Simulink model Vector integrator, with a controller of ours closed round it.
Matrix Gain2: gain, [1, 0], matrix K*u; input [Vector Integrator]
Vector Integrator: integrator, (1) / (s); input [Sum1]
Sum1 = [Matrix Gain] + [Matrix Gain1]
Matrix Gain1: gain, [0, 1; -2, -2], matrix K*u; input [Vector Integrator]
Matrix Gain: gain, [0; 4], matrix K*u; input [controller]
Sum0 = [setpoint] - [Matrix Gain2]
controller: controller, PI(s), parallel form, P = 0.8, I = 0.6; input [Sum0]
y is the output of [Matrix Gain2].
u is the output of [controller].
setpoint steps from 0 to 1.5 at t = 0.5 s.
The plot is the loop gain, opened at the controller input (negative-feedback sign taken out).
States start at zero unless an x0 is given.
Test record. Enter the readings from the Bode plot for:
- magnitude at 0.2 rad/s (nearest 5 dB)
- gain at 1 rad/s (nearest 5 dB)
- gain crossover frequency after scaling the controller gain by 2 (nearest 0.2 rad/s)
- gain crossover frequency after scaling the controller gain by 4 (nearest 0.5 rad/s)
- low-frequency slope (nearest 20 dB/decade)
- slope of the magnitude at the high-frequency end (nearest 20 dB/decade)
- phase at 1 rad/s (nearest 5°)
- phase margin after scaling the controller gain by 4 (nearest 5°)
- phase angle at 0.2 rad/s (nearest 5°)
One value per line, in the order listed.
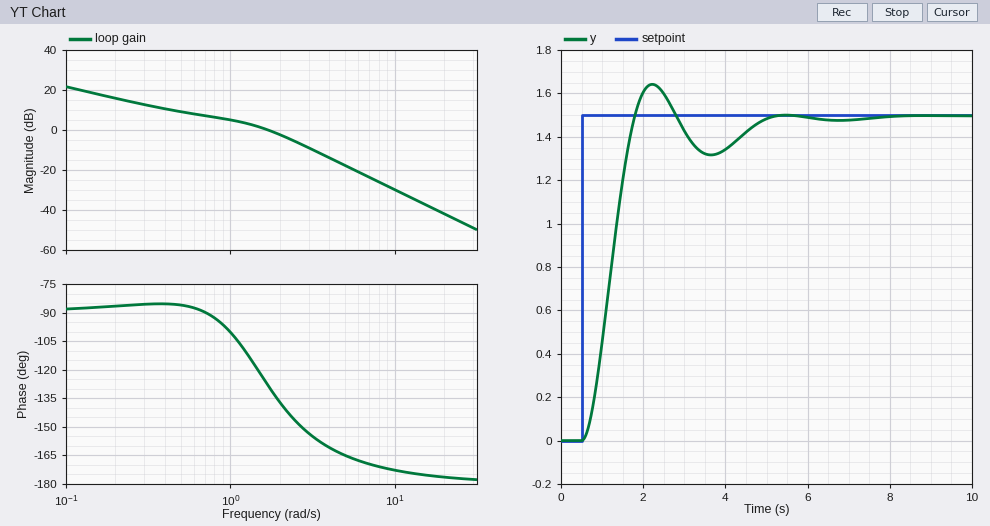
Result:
15 dB
5 dB
2.6 rad/s
3.5 rad/s
-20 dB/decade
-40 dB/decade
-100°
20°
-85°
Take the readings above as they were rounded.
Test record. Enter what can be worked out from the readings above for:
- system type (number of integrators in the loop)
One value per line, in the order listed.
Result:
1
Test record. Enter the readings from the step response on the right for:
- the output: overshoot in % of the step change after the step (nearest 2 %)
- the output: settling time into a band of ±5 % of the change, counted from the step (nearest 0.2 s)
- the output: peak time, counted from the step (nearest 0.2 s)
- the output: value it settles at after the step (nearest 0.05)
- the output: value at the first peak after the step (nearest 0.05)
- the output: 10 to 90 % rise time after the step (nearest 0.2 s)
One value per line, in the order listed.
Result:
10 %
4.0 s
1.8 s
1.50
1.65
0.8 s
